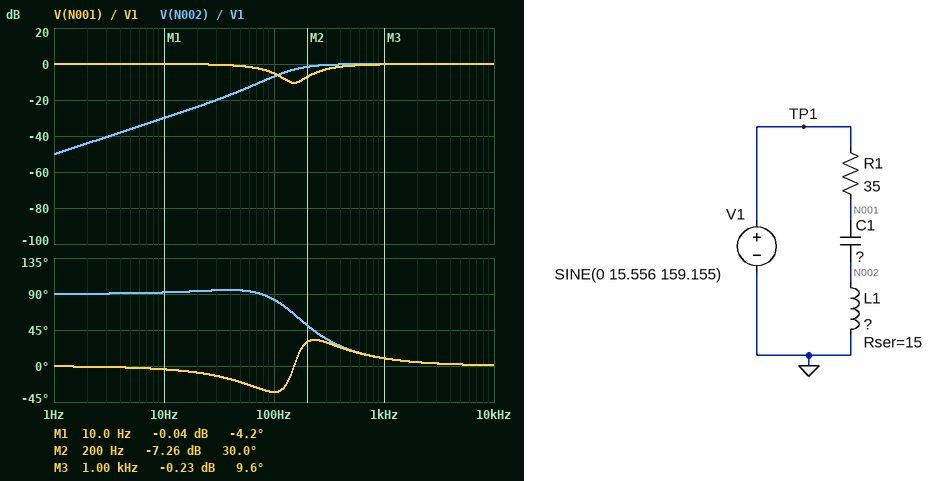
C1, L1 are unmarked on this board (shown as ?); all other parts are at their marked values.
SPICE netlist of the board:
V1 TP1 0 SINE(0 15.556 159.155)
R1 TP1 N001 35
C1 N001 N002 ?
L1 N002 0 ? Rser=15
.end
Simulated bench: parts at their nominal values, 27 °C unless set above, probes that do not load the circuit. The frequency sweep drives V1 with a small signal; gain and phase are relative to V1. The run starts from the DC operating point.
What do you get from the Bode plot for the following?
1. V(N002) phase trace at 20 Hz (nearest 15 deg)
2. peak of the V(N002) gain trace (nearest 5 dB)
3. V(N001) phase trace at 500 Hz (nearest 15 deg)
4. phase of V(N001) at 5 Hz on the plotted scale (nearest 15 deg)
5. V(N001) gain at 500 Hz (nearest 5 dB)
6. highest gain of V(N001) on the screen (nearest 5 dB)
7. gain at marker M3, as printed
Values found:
90 deg
0 dB
15 deg
0 deg
0 dB
0 dB
-0.23 dB
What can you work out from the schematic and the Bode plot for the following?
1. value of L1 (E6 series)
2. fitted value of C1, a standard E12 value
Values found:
33 mH
33 µF
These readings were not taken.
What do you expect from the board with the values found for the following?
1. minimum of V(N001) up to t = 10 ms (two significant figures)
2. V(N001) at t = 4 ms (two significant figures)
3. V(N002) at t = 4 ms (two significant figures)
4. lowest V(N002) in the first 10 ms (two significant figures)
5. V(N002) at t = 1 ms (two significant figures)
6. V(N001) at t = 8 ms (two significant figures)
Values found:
-4.5 V
-3.3 V
-10 V
-11 V
7.1 V
4.5 V
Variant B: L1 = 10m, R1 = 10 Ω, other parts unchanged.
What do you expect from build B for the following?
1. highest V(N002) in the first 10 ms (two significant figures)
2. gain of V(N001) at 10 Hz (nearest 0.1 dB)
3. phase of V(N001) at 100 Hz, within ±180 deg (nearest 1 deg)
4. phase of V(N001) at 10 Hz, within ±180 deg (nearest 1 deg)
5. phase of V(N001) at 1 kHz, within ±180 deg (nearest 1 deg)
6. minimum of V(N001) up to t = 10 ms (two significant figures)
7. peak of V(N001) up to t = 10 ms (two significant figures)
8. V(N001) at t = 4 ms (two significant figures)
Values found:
8.7 V
0 dB
-11 deg
-1 deg
9 deg
-12 V
13 V
-7.0 V
